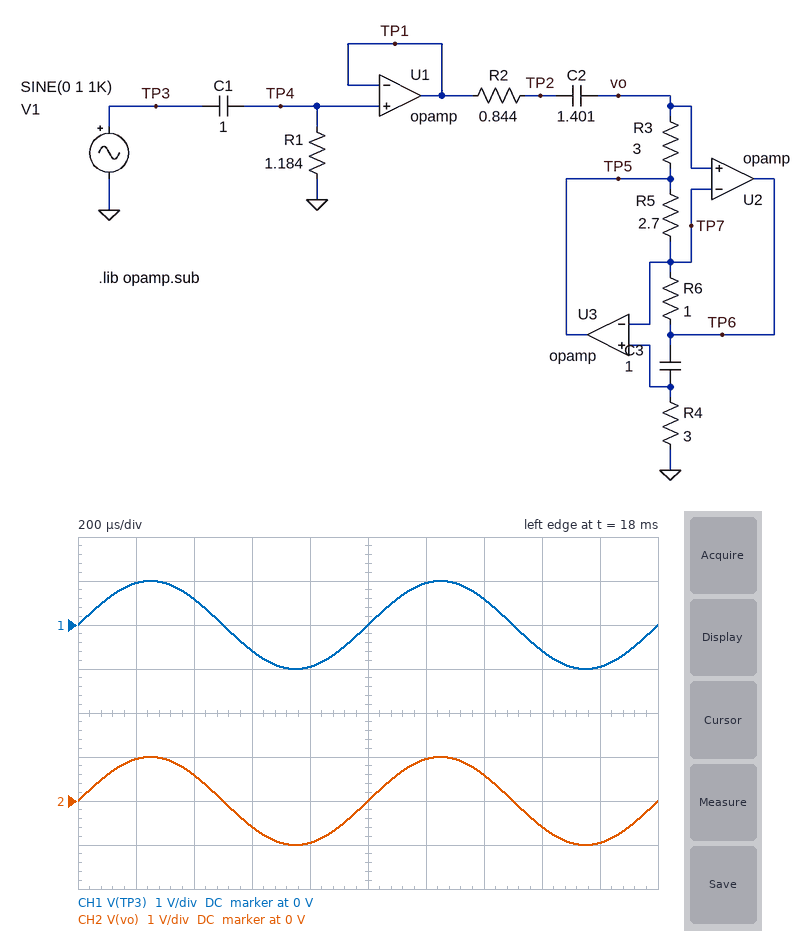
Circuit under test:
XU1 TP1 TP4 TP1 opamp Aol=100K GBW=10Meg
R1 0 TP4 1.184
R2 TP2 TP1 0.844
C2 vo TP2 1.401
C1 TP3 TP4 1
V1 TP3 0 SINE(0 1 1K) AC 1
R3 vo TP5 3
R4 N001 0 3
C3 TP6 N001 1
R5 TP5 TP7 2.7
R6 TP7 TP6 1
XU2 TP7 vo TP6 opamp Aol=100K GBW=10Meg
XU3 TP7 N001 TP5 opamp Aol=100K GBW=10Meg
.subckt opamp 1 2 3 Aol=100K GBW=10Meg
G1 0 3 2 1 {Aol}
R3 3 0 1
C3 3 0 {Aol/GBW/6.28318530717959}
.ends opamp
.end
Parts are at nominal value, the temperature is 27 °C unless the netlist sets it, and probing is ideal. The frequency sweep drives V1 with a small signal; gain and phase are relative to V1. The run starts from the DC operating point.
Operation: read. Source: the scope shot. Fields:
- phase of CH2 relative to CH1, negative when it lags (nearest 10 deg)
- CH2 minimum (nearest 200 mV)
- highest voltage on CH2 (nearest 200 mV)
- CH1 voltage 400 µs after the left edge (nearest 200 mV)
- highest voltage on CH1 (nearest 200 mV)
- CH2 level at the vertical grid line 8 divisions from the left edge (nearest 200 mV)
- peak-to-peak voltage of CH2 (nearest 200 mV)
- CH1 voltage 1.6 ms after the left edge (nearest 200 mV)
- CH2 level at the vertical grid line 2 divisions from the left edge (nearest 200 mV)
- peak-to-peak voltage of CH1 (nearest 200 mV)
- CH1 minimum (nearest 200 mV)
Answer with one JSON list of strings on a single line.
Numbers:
["0 deg", "-1.0 V", "1.0 V", "600 mV", "1.0 V", "-600 mV", "2.0 V", "-600 mV", "600 mV", "2.0 V", "-1.0 V"]
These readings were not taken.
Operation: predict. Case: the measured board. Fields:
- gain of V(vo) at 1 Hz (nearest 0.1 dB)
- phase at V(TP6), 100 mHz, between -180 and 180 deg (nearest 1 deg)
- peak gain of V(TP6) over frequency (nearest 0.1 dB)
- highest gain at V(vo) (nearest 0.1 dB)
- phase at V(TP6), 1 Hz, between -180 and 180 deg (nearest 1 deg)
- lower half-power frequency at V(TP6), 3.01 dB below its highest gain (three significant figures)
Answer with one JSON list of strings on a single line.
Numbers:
["0 dB", "67 deg", "1.4 dB", "0 dB", "7 deg", "65.2 mHz"]
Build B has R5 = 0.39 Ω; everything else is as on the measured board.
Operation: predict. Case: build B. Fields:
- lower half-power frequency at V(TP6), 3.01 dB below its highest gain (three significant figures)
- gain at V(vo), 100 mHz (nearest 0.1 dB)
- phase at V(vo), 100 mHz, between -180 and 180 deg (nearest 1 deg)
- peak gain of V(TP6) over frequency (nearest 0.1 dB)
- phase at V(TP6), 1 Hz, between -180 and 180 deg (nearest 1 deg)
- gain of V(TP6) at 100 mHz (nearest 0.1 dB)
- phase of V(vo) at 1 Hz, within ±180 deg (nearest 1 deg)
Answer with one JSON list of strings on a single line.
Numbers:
["25.8 mHz", "-3.8 dB", "57 deg", "6.5 dB", "5 deg", "-2.7 dB", "8 deg"]
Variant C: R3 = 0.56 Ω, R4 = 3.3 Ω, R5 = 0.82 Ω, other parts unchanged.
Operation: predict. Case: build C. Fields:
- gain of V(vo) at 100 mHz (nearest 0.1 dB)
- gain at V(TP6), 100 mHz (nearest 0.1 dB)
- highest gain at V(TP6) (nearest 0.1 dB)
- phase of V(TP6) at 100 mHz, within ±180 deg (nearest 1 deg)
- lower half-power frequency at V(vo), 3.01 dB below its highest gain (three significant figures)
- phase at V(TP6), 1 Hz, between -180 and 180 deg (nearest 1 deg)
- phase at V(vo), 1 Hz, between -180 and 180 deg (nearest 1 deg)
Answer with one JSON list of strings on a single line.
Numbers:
["-0.4 dB", "0.5 dB", "0.7 dB", "99 deg", "82.7 mHz", "8 deg", "11 deg"]
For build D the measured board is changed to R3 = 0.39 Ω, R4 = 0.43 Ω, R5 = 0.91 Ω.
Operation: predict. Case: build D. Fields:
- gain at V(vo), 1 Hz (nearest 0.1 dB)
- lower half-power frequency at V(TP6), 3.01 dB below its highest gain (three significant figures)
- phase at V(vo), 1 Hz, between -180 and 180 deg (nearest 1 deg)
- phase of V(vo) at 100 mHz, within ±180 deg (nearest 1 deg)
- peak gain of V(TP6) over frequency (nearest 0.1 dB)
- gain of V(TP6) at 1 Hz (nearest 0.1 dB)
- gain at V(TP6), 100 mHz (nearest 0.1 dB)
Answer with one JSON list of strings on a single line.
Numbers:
["-1.4 dB", "418 mHz", "47 deg", "-166 deg", "0 dB", "-0.8 dB", "-14.0 dB"]
